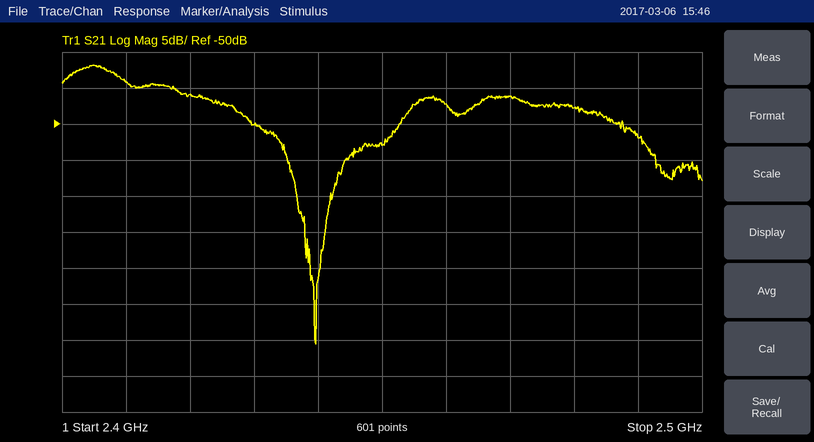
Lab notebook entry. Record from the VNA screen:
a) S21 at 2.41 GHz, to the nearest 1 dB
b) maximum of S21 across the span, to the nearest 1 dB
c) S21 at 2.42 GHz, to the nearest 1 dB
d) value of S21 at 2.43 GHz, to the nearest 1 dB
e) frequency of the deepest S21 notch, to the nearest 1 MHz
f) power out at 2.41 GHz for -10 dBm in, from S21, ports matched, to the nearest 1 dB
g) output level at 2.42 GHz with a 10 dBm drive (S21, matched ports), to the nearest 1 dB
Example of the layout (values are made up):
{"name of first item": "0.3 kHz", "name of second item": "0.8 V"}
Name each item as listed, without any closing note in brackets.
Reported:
{"S21 at 2.41 GHz, to the nearest 1 dB": "-44 dB", "maximum of S21 across the span, to the nearest 1 dB": "-42 dB", "S21 at 2.42 GHz, to the nearest 1 dB": "-46 dB", "value of S21 at 2.43 GHz, to the nearest 1 dB": "-50 dB", "frequency of the deepest S21 notch, to the nearest 1 MHz": "2.440 GHz", "power out at 2.41 GHz for -10 dBm in, from S21, ports matched, to the nearest 1 dB": "-54 dBm", "output level at 2.42 GHz with a 10 dBm drive (S21, matched ports), to the nearest 1 dB": "-36 dBm"}
